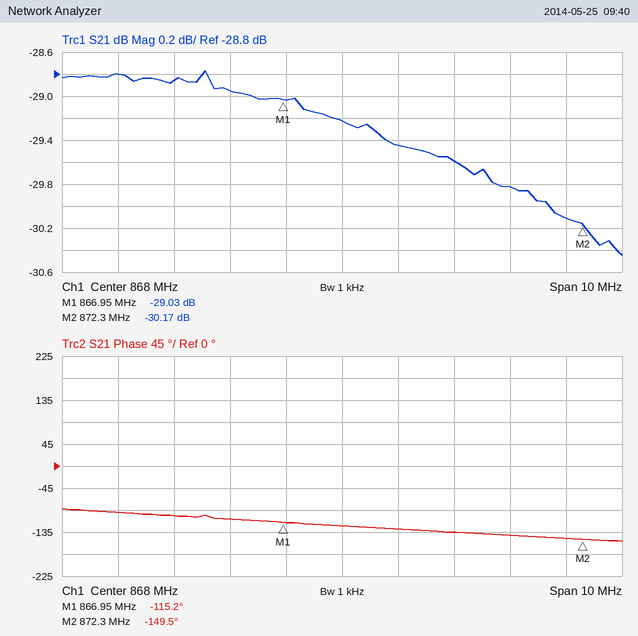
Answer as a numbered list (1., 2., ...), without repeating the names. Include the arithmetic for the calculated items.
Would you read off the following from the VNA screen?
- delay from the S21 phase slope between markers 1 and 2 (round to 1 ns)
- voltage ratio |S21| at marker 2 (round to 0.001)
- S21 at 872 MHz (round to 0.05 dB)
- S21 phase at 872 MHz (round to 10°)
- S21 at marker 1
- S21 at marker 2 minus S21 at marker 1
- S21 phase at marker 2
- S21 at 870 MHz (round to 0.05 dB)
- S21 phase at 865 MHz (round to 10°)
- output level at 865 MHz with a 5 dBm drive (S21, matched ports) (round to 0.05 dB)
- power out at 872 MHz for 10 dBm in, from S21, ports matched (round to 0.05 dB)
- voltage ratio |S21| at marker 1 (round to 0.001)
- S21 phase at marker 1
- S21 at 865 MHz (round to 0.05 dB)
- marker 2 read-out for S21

1. −(-149.5° − (-115.2°))/(360° × 5.35 MHz) ≈ 18 ns
2. 10^(-30.17/20) ≈ 0.031
3. -30.10 dB
4. -150°
5. -29.03 dB
6. -30.17 − (-29.03) = -1.14 dB
7. -149.5°
8. -29.60 dB
9. -100°
10. 5 dBm + (-28.85 dB) = -23.85 dBm
11. 10 dBm + (-30.10 dB) = -20.10 dBm
12. 10^(-29.03/20) ≈ 0.035
13. -115.2°
14. -28.85 dB
15. -30.17 dB
